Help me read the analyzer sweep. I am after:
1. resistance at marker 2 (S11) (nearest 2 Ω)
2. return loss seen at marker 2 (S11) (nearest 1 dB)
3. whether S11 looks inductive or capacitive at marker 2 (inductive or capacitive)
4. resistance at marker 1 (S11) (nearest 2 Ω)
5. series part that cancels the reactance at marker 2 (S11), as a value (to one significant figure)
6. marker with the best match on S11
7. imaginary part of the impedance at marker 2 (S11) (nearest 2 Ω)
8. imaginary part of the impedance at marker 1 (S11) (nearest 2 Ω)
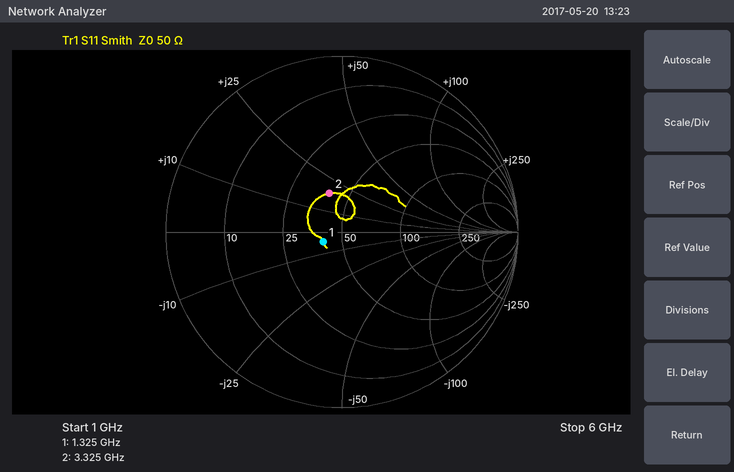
40 Ω
13 dB
inductive
40 Ω
3 pF
marker 1
+18 Ω
-4 Ω
